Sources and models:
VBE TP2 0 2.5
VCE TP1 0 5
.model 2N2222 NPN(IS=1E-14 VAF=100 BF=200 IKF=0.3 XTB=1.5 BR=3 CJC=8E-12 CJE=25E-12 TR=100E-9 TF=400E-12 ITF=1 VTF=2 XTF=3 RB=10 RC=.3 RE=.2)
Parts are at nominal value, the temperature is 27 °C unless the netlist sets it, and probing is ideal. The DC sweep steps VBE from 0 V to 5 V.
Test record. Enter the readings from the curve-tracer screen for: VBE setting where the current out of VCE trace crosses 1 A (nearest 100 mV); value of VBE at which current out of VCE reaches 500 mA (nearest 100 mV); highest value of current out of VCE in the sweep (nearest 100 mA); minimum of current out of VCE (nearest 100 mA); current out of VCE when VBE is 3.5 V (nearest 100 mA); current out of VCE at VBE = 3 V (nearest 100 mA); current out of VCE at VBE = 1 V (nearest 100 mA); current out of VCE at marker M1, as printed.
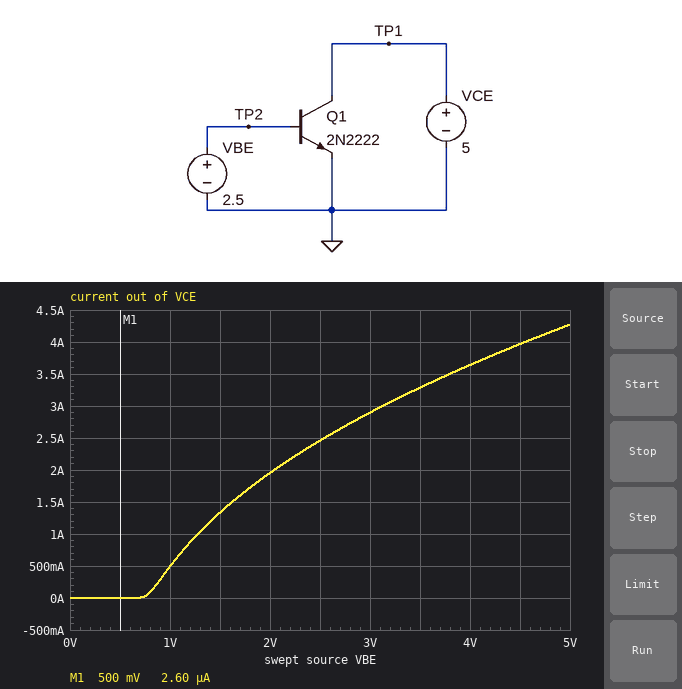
1.3 V
1.0 V
4.3 A
0 A
3.3 A
2.9 A
500 mA
2.60 µA
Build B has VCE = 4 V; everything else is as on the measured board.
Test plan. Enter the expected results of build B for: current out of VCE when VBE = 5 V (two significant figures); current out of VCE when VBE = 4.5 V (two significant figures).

4.2 A
3.9 A
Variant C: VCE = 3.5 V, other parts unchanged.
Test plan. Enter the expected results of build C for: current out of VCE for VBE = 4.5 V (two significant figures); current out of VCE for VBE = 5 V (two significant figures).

3.9 A
4.2 A
